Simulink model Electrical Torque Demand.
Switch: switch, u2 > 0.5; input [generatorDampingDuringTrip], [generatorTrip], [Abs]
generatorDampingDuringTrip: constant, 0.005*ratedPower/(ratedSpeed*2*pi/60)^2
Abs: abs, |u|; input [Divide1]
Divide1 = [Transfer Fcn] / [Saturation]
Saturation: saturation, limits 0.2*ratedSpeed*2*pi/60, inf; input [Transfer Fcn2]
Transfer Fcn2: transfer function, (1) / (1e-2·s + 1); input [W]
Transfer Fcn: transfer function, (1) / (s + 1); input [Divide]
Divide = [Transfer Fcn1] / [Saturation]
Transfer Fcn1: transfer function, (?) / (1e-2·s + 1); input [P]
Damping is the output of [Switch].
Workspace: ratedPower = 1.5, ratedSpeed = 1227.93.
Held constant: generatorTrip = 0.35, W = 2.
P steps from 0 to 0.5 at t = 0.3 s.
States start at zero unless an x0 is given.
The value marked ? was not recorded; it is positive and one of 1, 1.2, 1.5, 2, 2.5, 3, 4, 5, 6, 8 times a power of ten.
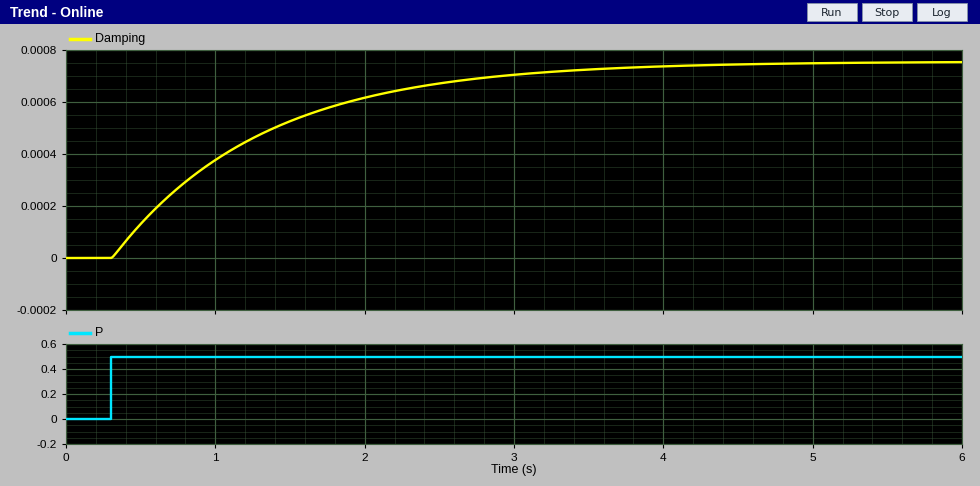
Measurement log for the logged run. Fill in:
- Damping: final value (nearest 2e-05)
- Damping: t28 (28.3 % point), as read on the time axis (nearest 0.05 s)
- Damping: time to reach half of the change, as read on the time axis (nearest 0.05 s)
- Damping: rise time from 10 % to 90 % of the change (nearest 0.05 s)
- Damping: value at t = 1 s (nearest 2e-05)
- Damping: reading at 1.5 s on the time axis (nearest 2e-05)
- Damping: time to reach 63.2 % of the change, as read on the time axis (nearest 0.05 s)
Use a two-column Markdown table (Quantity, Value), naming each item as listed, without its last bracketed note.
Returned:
| Quantity | Value |
|---|---|
| Damping: final value | 0.00076 |
| Damping: t28 (28.3 % point), as read on the time axis | 0.65 s |
| Damping: time to reach half of the change, as read on the time axis | 1.00 s |
| Damping: rise time from 10 % to 90 % of the change | 2.20 s |
| Damping: value at t = 1 s | 0.00038 |
| Damping: reading at 1.5 s on the time axis | 0.00052 |
| Damping: time to reach 63.2 % of the change, as read on the time axis | 1.30 s |
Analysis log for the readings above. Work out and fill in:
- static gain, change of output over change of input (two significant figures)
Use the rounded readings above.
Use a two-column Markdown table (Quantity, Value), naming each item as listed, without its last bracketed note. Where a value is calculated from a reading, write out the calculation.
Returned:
| Quantity | Value |
|---|---|
| static gain, change of output over change of input | (0.00076 - 0) / (0.5 - 0) = 0.0015 |
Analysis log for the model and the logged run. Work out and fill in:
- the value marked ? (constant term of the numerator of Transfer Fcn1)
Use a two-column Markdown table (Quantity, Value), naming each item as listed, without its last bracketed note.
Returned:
| Quantity | Value |
|---|---|
| the value marked ? | 1 |
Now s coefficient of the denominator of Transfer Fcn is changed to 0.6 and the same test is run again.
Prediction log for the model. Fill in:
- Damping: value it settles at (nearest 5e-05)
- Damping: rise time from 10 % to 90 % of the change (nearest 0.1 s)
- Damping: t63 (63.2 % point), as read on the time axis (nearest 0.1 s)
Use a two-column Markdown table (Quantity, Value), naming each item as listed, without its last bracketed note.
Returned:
| Quantity | Value |
|---|---|
| Damping: value it settles at | 0.00075 |
| Damping: rise time from 10 % to 90 % of the change | 1.3 s |
| Damping: t63 (63.2 % point), as read on the time axis | 0.9 s |
